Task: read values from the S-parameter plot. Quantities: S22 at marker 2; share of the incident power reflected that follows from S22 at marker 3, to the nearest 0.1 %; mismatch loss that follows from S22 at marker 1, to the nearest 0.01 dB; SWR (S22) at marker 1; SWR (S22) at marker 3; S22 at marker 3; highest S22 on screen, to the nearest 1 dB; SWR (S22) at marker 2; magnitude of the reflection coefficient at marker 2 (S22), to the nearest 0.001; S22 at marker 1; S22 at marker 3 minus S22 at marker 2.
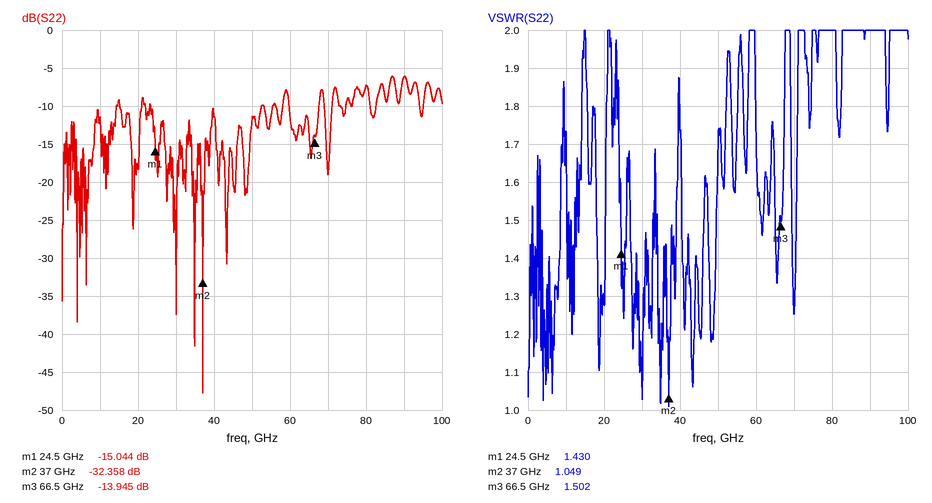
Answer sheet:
-32.358 dB
4.0 %
0.14 dB
1.430
1.502
-13.945 dB
-6 dB
1.049
0.024
-15.044 dB
18.413 dB
